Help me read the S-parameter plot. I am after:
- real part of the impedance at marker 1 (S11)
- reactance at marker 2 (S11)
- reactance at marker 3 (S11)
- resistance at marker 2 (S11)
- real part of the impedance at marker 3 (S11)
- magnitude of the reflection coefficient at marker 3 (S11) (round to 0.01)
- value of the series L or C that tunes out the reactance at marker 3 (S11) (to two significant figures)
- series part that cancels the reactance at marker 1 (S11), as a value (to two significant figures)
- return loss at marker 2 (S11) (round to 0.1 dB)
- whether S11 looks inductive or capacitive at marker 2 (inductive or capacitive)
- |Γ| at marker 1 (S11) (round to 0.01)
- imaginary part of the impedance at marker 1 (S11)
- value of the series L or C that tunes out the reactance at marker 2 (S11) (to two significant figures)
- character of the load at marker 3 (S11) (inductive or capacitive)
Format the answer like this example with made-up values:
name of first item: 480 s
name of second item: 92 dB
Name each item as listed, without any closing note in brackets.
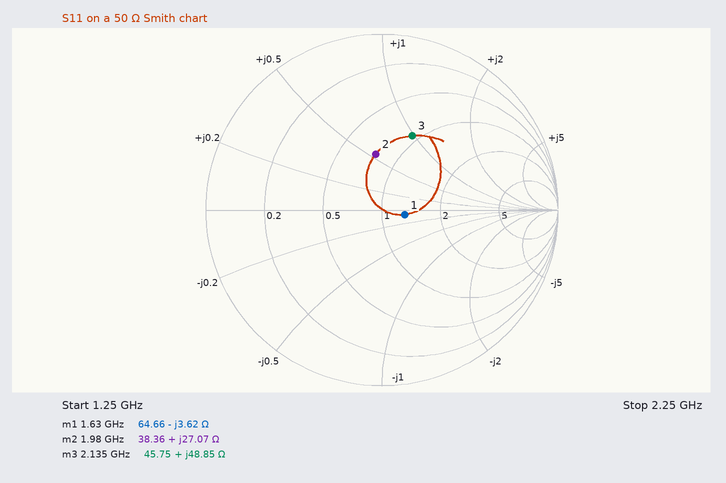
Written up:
real part of the impedance at marker 1: 64.66 Ω
reactance at marker 2: +27.07 Ω
reactance at marker 3: +48.85 Ω
resistance at marker 2: 38.36 Ω
real part of the impedance at marker 3: 45.75 Ω
magnitude of the reflection coefficient at marker 3 (S11): 0.46
value of the series L or C that tunes out the reactance at marker 3 (S11): 1.5 pF
series part that cancels the reactance at marker 1 (S11), as a value: 350 pH
return loss at marker 2 (S11): 9.9 dB
whether S11 looks inductive or capacitive at marker 2: inductive
|Γ| at marker 1 (S11): 0.13
imaginary part of the impedance at marker 1: -3.62 Ω
value of the series L or C that tunes out the reactance at marker 2 (S11): 3.0 pF
character of the load at marker 3 (S11): inductive
